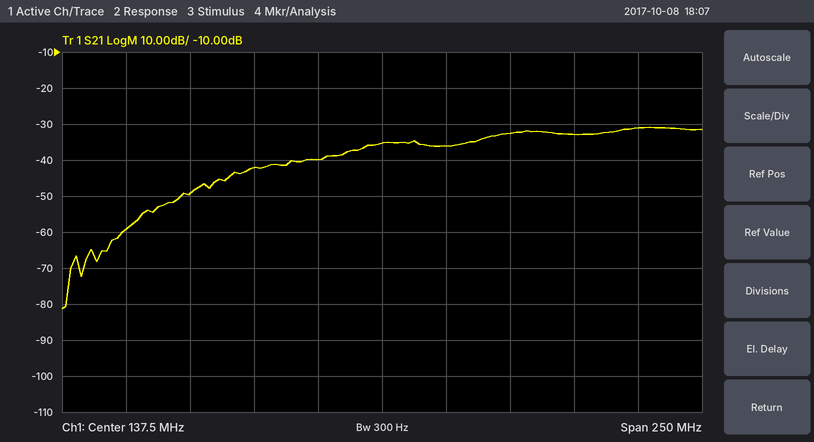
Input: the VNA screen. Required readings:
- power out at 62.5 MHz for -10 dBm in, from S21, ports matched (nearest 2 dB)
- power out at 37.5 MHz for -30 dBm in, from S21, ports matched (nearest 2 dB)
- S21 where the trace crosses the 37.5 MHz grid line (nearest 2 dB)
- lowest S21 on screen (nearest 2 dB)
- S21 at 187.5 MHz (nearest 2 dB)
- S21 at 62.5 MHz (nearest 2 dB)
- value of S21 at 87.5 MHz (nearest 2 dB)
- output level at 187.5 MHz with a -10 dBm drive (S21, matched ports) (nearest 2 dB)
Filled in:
-60 dBm
-90 dBm
-60 dB
-82 dB
-32 dB
-50 dB
-42 dB
-42 dBm
